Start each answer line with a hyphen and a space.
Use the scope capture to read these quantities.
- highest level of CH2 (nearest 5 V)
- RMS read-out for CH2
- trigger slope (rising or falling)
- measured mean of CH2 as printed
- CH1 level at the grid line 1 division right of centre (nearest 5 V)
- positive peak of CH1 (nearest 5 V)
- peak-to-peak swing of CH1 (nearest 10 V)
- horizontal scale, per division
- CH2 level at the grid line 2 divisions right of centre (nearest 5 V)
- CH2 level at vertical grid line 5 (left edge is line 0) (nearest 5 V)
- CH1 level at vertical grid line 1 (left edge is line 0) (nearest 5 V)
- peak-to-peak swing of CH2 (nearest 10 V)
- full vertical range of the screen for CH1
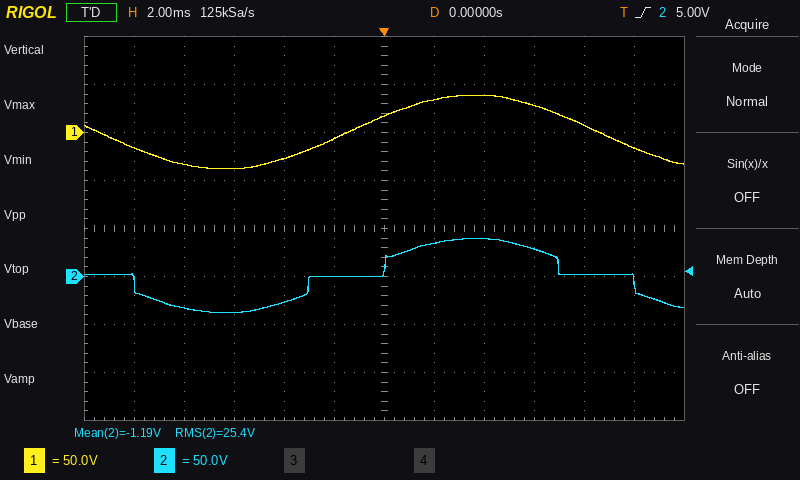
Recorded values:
- 40 V
- 25.4 V
- rising
- -1.19 V
- 35 V
- 40 V
- 80 V
- 2 ms
- 40 V
- 0 V
- -15 V
- 80 V
- 400 V
